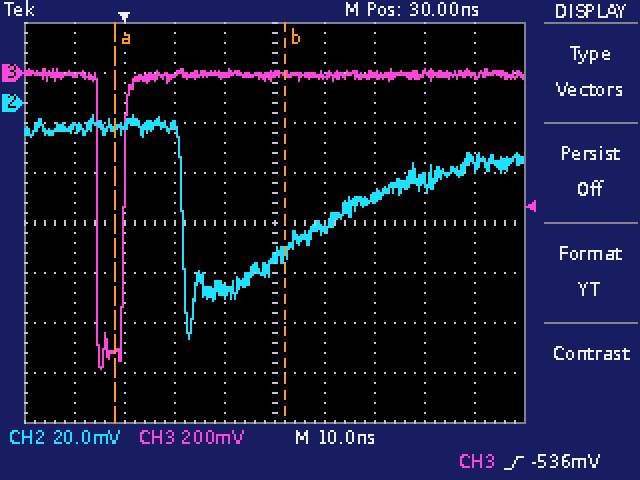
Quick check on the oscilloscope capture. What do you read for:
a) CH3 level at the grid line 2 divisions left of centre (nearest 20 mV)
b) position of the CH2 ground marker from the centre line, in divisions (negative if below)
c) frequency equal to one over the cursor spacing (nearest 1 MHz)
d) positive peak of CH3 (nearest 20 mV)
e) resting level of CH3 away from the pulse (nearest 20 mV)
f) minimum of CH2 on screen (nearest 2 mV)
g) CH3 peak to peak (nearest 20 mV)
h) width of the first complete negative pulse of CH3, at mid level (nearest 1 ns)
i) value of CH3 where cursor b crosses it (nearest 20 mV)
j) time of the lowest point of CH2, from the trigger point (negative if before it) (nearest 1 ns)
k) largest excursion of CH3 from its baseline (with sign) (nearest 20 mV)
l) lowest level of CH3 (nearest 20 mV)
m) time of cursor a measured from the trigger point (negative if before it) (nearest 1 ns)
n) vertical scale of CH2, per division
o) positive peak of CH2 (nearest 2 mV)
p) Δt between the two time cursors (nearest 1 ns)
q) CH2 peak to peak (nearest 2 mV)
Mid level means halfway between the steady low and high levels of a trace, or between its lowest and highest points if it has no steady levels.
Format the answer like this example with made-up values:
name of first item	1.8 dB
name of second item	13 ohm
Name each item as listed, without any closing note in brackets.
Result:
CH3 level at the grid line 2 divisions left of centre	0 mV
position of the CH2 ground marker from the centre line, in divisions	+2.4 div
frequency equal to one over the cursor spacing	29 MHz
positive peak of CH3	20 mV
resting level of CH3 away from the pulse	0 mV
minimum of CH2 on screen	-94 mV
CH3 peak to peak	1.20 V
width of the first complete negative pulse of CH3, at mid level	5 ns
value of CH3 where cursor b crosses it	0 mV
time of the lowest point of CH2, from the trigger point (negative if before it)	+13 ns
largest excursion of CH3 from its baseline (with sign)	-1.18 V
lowest level of CH3	-1.18 V
time of cursor a measured from the trigger point (negative if before it)	-2 ns
vertical scale of CH2, per division	20 mV
positive peak of CH2	-4 mV
Δt between the two time cursors	34 ns
CH2 peak to peak	90 mV
